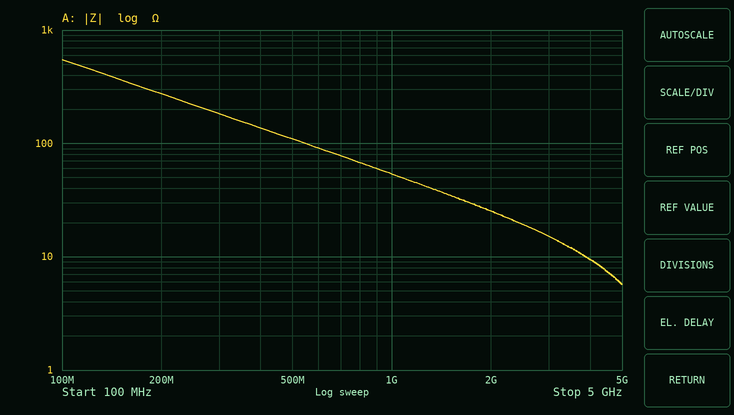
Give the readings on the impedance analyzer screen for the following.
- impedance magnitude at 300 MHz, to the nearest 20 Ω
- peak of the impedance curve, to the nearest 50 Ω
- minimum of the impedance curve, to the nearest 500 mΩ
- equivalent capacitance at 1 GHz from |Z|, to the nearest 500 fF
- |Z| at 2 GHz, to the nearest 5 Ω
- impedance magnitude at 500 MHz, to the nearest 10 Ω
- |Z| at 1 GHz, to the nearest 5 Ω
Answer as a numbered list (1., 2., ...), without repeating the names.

1. 180 Ω
2. 550 Ω
3. 5.5 Ω
4. 3.0 pF
5. 25 Ω
6. 110 Ω
7. 55 Ω
